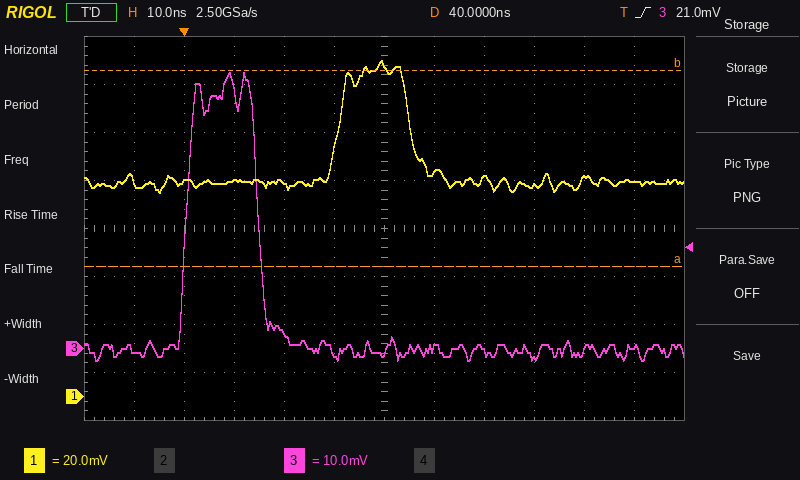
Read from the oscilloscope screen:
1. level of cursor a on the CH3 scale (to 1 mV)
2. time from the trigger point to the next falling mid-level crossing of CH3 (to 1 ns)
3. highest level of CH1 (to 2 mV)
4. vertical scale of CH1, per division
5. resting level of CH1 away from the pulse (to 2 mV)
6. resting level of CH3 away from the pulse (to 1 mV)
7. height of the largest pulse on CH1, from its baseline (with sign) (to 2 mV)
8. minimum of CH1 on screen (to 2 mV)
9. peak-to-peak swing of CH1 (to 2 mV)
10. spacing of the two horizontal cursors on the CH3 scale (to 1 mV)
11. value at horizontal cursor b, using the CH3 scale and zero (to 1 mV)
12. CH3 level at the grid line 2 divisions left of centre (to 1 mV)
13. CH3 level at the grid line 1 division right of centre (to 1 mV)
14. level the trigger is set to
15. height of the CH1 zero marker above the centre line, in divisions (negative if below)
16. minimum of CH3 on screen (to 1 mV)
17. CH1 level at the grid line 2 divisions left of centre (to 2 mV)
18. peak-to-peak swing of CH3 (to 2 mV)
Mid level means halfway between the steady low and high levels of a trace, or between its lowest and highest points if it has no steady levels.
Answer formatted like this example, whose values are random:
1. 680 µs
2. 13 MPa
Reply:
1. 17 mV
2. 15 ns
3. 140 mV
4. 20 mV
5. 90 mV
6. 0 mV
7. +50 mV
8. 84 mV
9. 56 mV
10. 41 mV
11. 58 mV
12. 3 mV
13. 0 mV
14. 21.0 mV
15. -3.5 div
16. -2 mV
17. 88 mV
18. 60 mV
